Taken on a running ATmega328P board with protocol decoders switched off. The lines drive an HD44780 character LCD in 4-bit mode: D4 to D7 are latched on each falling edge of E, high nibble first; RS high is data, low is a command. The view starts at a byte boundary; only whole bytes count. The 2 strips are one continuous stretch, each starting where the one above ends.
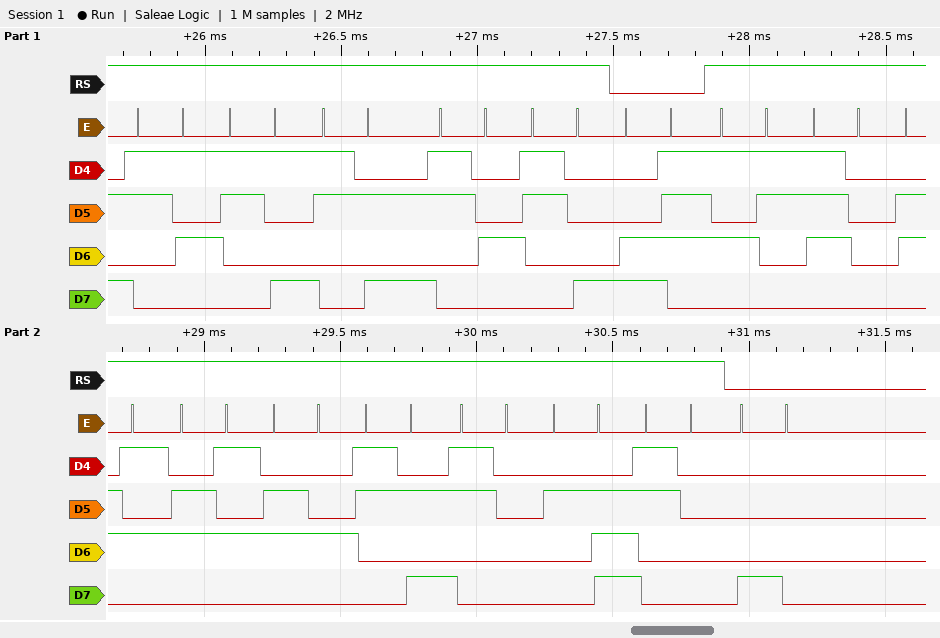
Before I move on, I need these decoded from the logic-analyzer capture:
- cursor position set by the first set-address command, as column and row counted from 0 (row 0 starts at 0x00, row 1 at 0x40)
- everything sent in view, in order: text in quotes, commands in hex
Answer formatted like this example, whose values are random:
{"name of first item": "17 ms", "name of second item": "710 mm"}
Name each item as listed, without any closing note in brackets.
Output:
{"cursor position set by the first set-address command, as column and row counted from 0": "column 7, row 1", "everything sent in view, in order: text in quotes, commands in hex": "\"59:48\" 0xC7 \"Speed:0.0\" 0x80"}
